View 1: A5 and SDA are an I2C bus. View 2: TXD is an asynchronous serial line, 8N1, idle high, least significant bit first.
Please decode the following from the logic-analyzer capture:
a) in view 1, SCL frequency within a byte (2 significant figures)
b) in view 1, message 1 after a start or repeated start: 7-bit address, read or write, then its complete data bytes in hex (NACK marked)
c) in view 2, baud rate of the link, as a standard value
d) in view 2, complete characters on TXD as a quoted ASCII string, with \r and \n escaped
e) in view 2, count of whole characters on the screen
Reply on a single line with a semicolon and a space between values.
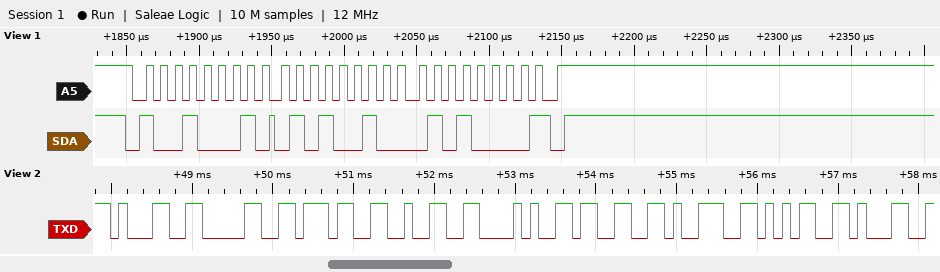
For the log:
100 kHz; 0x48 read: 52 50 NACK; 9600 baud; "1072(3951"; 9
